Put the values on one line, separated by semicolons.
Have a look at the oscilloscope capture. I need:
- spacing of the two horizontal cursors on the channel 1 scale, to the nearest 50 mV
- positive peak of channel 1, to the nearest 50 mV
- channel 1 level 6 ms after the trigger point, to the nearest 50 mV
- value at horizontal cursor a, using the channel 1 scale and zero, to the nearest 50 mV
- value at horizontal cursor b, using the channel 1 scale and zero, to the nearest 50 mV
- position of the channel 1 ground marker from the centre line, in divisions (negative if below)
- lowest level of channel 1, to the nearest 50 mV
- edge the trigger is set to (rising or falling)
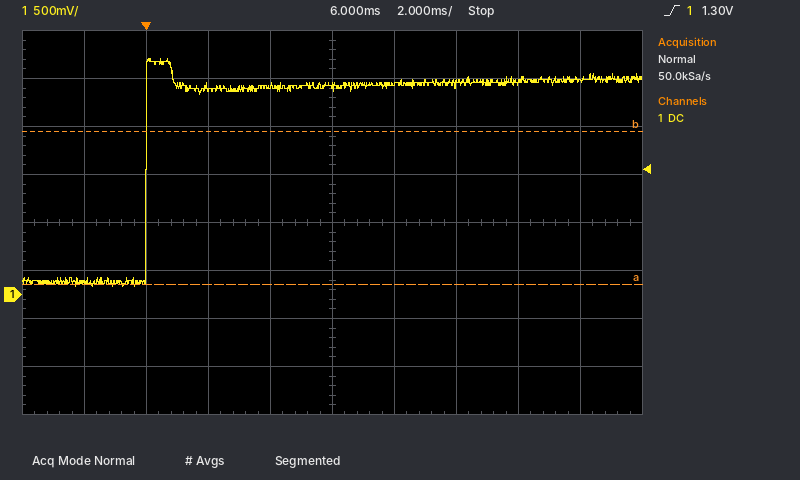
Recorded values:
1.60 V; 2.45 V; 2.15 V; 100 mV; 1.70 V; -1.5 div; 100 mV; rising
